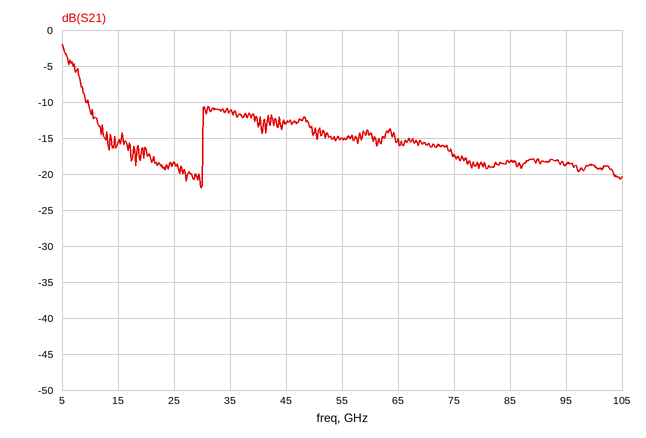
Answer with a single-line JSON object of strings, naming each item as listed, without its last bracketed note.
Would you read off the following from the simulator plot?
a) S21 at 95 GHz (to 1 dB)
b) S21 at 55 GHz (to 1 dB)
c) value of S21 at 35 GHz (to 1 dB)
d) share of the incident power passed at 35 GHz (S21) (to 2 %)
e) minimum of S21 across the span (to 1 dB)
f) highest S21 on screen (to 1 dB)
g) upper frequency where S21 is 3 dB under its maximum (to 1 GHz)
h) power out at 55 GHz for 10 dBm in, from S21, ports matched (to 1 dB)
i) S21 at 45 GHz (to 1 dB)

{"S21 at 95 GHz": "-19 dB", "S21 at 55 GHz": "-15 dB", "value of S21 at 35 GHz": "-11 dB", "share of the incident power passed at 35 GHz (S21)": "8 %", "minimum of S21 across the span": "-22 dB", "highest S21 on screen": "-2 dB", "upper frequency where S21 is 3 dB under its maximum": "7 GHz", "power out at 55 GHz for 10 dBm in, from S21, ports matched": "-5 dBm", "S21 at 45 GHz": "-13 dB"}
